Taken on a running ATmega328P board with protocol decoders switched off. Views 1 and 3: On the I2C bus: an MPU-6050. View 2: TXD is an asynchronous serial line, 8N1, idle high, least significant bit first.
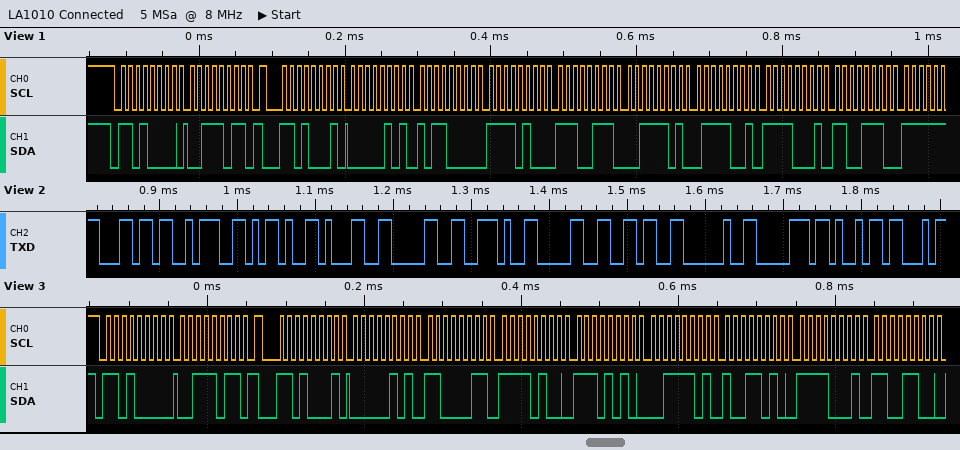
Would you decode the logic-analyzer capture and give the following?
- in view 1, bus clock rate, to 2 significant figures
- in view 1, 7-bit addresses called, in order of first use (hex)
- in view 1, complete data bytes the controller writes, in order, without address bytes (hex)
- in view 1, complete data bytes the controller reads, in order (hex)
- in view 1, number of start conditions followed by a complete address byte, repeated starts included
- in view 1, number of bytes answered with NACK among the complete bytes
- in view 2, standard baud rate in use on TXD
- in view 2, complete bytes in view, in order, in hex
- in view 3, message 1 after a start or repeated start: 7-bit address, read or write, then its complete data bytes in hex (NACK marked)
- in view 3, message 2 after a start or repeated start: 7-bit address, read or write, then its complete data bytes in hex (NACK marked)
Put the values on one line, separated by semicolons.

100 kHz; 0x68; 3B; 05 B0 F4 E7 3D 79 F1 CE; 2; 0; 115200 baud; 6C 3A 2D 31 30 2E 30 36 20 70 69; 0x68 write: 3B; 0x68 read: 05 C3 F4 EA 3D 9A F1 CC
